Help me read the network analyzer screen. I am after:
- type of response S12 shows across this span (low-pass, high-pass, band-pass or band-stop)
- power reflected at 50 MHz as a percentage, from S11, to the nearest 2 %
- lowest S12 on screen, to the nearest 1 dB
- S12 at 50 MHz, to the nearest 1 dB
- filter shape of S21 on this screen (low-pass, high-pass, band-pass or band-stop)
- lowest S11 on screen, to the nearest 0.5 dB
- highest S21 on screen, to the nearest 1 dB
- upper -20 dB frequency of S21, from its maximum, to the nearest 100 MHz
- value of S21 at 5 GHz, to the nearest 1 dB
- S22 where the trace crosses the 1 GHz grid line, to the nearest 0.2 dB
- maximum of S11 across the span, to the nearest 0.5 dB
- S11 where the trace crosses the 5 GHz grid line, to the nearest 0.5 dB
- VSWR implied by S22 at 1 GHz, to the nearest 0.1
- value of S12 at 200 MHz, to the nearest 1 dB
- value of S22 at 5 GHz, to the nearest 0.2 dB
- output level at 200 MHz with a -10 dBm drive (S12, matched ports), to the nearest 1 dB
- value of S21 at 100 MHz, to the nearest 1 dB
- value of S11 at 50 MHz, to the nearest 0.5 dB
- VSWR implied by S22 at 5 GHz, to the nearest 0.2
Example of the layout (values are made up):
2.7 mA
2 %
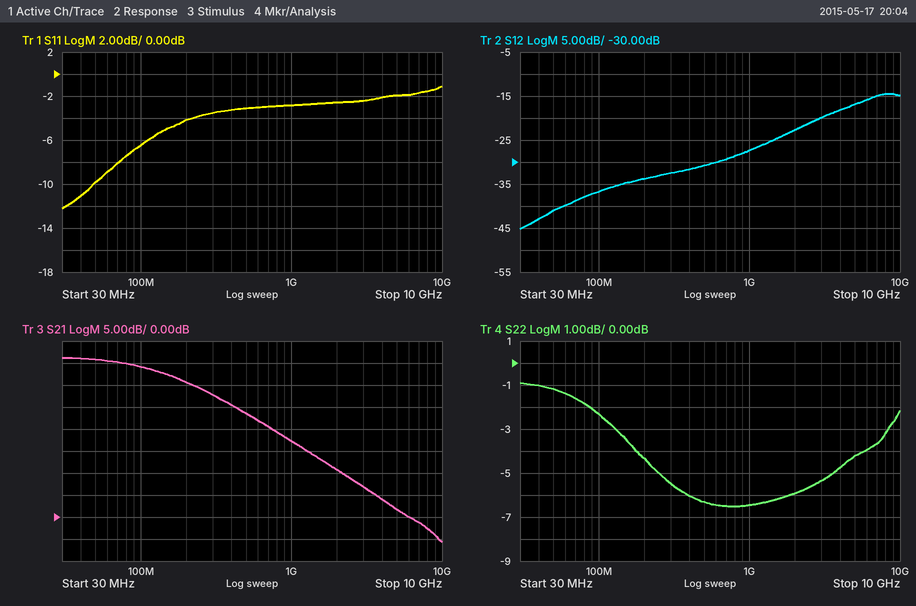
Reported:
high-pass
10 %
-45 dB
-41 dB
low-pass
-12.0 dB
36 dB
1.1 GHz
2 dB
-6.4 dB
-1.0 dB
-2.0 dB
2.8
-34 dB
-4.2 dB
-44 dBm
34 dB
-10.0 dB
4.2
